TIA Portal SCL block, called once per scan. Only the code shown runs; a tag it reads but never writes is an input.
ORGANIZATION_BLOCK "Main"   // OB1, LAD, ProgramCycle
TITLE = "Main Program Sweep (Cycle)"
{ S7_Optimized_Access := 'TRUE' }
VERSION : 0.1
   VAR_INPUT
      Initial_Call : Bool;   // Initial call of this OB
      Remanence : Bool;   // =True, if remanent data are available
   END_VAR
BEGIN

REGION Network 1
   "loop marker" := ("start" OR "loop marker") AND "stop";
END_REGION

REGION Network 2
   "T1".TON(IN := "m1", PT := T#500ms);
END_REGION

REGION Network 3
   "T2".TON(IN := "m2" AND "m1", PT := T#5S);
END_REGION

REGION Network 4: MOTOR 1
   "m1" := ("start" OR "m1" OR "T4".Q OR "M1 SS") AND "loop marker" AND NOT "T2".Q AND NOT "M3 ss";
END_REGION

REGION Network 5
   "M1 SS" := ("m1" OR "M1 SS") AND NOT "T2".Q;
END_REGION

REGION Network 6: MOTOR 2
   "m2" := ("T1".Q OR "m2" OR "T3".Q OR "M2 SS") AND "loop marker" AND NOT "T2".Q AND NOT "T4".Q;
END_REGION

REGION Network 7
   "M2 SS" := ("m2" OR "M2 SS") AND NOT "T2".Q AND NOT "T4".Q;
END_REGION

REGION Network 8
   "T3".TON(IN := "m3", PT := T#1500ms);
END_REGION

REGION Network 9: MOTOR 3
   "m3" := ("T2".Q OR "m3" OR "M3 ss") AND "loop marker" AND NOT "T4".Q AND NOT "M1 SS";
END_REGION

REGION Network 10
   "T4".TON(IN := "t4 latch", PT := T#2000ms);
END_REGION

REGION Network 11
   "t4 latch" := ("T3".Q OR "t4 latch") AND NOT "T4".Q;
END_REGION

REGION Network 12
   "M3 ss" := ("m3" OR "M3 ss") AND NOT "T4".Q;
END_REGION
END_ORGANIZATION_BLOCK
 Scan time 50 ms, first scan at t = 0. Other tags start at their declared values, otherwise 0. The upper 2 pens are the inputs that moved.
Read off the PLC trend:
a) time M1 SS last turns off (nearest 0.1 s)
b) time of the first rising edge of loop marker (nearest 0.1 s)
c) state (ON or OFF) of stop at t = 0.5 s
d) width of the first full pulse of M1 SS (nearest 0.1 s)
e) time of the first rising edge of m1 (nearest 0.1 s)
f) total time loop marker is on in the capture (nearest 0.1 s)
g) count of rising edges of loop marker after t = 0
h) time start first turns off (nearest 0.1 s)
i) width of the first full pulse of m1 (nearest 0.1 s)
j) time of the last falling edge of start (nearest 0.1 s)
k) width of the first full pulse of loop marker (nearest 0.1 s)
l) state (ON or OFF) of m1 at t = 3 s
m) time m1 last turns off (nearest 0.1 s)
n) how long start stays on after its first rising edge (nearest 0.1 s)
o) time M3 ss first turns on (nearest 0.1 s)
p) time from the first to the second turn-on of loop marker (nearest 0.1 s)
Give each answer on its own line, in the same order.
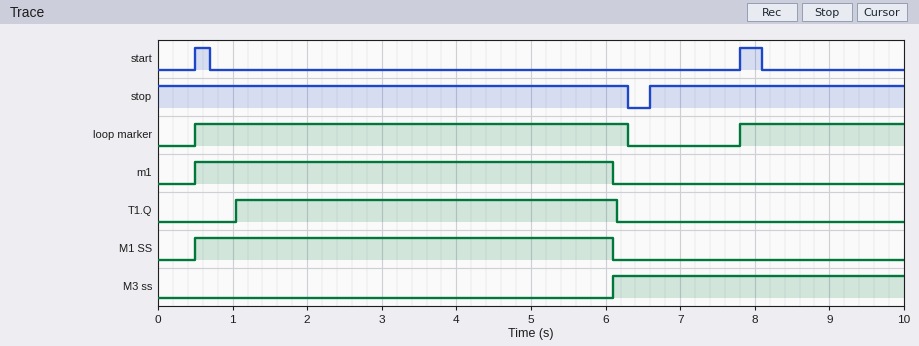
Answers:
6.1 s
0.5 s
ON
5.6 s
0.5 s
8.0 s
2
0.7 s
5.6 s
8.1 s
5.8 s
ON
6.1 s
0.2 s
6.1 s
7.3 s
